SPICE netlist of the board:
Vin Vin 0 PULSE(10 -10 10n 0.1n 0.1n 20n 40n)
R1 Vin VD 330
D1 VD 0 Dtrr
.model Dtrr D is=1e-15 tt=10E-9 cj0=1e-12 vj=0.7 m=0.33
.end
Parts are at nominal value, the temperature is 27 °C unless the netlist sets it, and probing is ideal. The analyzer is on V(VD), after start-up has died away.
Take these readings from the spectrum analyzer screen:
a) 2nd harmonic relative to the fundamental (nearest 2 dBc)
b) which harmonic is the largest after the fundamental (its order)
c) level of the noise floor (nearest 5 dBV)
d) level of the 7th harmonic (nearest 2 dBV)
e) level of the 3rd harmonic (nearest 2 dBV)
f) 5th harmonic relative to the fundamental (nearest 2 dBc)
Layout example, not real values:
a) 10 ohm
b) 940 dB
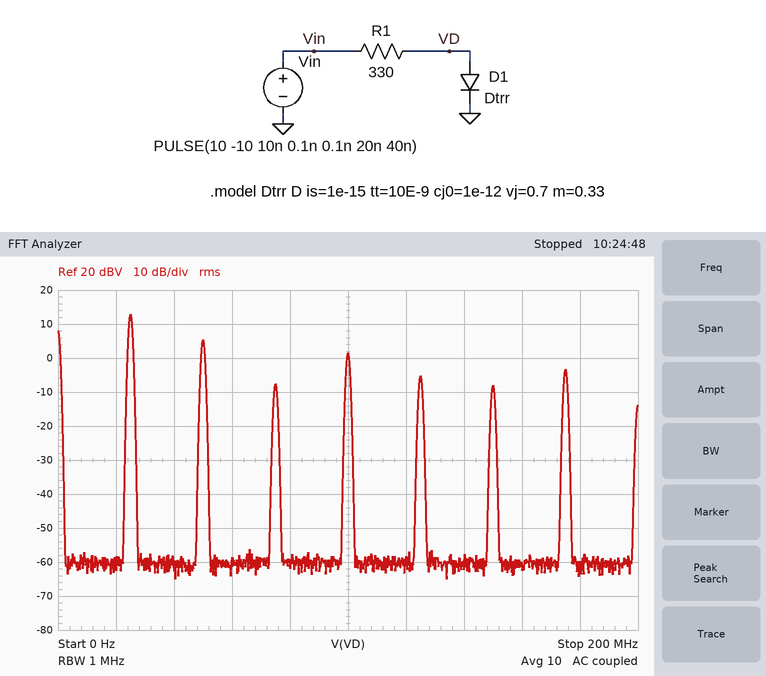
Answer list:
a) -8 dBc
b) 2
c) -60 dBV
d) -4 dBV
e) -8 dBV
f) -18 dBc
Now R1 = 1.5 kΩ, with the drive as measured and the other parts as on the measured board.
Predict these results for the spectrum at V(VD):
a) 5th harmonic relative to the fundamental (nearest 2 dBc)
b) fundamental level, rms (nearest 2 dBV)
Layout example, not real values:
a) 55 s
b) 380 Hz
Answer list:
a) -16 dBc
b) 12 dBV
